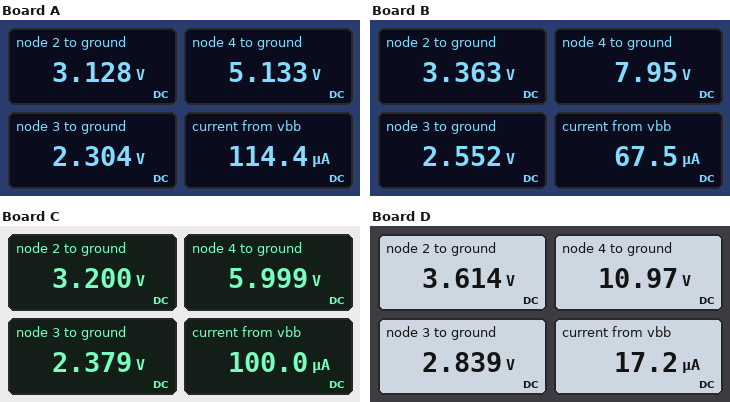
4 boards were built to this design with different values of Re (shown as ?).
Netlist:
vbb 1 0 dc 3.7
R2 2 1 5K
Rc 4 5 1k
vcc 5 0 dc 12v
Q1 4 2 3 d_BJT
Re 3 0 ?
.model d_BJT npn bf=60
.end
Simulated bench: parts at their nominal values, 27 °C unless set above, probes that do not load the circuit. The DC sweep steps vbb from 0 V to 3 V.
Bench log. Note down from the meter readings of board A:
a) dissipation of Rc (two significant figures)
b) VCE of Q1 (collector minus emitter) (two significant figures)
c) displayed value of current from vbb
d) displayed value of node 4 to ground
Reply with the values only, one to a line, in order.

47 mW
2.8 V
114.4 µA
5.133 V
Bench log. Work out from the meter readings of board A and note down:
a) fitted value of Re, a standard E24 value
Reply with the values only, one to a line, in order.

330 Ω
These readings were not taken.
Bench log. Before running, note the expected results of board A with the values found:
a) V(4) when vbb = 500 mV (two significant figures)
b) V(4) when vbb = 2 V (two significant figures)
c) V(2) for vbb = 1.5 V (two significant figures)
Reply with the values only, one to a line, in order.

12 V
9.1 V
1.4 V
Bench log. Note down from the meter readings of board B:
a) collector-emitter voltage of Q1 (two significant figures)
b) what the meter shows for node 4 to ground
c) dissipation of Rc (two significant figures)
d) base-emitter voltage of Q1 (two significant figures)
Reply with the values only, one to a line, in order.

5.4 V
7.95 V
16 mW
810 mV
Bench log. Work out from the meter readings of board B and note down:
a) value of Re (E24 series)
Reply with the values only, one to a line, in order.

620 Ω
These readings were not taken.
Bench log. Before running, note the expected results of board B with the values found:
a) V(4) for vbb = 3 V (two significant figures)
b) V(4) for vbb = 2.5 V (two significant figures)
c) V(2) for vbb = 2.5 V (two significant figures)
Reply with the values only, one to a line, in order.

8.9 V
9.6 V
2.3 V
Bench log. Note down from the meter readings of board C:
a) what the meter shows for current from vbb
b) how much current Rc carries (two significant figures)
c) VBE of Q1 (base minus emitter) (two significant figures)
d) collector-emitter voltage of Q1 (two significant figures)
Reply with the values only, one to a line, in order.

100.0 µA
6.0 mA
820 mV
3.6 V
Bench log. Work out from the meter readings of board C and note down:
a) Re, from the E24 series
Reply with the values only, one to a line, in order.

390 Ω
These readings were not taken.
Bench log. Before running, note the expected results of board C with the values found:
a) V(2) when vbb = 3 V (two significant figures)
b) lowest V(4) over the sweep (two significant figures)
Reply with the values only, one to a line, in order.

2.6 V
7.4 V
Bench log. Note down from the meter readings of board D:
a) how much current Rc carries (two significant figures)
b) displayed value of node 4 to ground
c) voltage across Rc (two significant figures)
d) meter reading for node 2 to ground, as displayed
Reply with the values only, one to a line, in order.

1.0 mA
10.97 V
1.0 V
3.614 V
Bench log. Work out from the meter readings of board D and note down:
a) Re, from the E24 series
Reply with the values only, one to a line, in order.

2.7 kΩ
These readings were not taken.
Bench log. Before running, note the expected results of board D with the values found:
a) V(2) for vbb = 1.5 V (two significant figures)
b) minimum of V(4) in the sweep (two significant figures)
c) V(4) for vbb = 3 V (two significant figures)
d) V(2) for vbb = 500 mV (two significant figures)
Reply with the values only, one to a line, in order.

1.5 V
11 V
11 V
500 mV
